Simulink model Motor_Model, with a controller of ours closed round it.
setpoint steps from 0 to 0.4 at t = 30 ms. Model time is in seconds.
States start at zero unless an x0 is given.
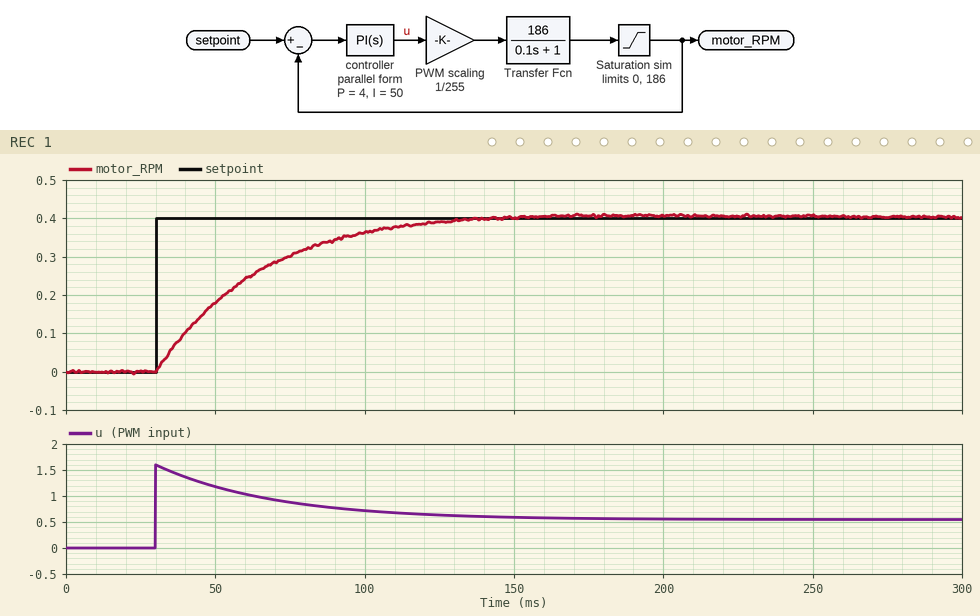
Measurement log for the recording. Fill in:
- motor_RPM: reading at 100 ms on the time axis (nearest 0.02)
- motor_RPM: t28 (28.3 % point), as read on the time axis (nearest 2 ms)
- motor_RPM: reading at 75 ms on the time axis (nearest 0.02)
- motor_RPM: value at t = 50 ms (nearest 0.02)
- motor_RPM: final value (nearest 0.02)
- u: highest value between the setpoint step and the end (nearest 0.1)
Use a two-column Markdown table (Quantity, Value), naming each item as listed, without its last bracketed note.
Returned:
| Quantity | Value |
|---|---|
| motor_RPM: reading at 100 ms on the time axis | 0.36 |
| motor_RPM: t28 (28.3 % point), as read on the time axis | 42 ms |
| motor_RPM: reading at 75 ms on the time axis | 0.30 |
| motor_RPM: value at t = 50 ms | 0.18 |
| motor_RPM: final value | 0.40 |
| u: highest value between the setpoint step and the end | 1.6 |
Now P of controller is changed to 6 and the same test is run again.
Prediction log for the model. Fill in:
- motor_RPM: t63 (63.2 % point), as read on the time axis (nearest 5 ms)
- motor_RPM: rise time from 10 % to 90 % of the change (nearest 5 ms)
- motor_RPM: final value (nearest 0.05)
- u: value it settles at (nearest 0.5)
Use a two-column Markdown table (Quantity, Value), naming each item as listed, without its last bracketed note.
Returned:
| Quantity | Value |
|---|---|
| motor_RPM: t63 (63.2 % point), as read on the time axis | 55 ms |
| motor_RPM: rise time from 10 % to 90 % of the change | 55 ms |
| motor_RPM: final value | 0.40 |
| u: value it settles at | 0.5 |
